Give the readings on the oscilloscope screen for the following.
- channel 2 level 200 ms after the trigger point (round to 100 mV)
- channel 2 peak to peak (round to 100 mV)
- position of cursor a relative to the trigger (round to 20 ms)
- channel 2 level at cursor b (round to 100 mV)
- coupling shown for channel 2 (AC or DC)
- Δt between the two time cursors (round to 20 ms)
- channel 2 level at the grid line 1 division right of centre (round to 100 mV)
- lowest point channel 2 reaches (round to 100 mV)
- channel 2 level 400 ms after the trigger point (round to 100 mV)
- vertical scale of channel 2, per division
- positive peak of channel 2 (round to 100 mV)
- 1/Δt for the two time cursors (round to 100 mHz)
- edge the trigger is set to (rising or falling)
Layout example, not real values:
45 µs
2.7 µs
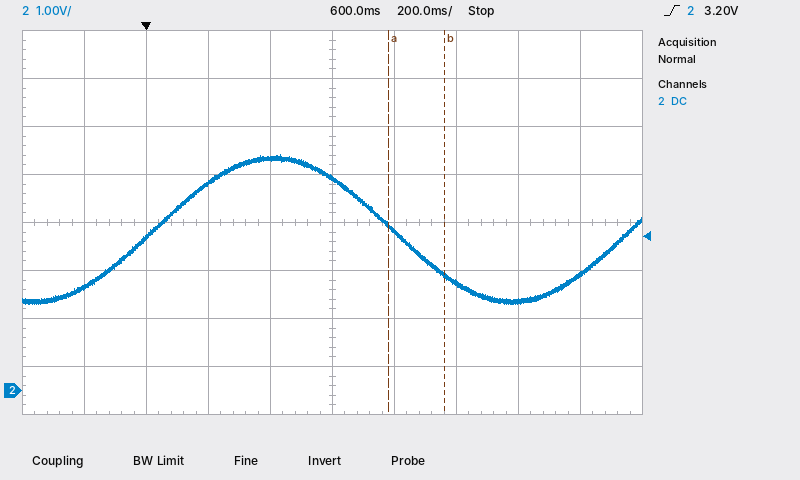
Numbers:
4.3 V
3.1 V
+780 ms
2.4 V
DC
180 ms
3.3 V
1.8 V
4.8 V
1 V
4.9 V
5.6 Hz
rising
